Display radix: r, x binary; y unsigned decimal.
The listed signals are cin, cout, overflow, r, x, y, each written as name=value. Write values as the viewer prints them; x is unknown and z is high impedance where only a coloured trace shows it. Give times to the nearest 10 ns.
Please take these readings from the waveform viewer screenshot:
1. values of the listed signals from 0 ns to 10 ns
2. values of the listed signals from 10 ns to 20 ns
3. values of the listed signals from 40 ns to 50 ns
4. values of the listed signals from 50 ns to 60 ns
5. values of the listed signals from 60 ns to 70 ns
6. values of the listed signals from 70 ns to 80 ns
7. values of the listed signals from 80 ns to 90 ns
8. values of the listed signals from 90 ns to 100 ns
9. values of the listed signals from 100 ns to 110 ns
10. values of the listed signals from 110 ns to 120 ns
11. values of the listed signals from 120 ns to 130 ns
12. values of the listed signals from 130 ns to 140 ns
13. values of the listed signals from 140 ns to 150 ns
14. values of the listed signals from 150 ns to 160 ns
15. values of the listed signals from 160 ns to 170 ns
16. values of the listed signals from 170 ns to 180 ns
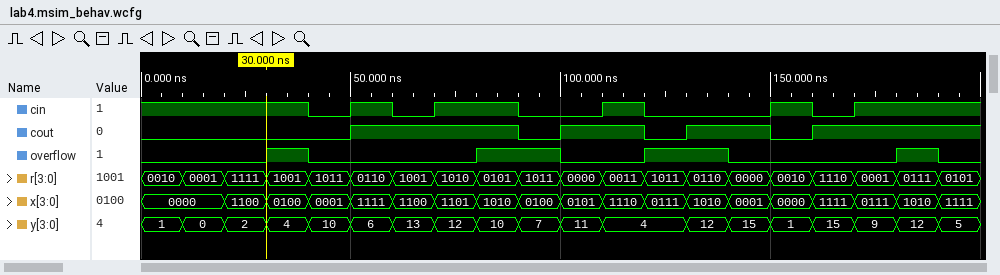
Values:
cin=1, cout=0, overflow=0, r=0010, x=0000, y=1
cin=1, cout=0, overflow=0, r=0001, x=0000, y=0
cin=0, cout=0, overflow=0, r=1011, x=0001, y=10
cin=1, cout=1, overflow=0, r=0110, x=1111, y=6
cin=0, cout=1, overflow=0, r=1001, x=1100, y=13
cin=1, cout=1, overflow=0, r=1010, x=1101, y=12
cin=1, cout=1, overflow=1, r=0101, x=1010, y=10
cin=0, cout=0, overflow=1, r=1011, x=0100, y=7
cin=0, cout=1, overflow=0, r=0000, x=0101, y=11
cin=1, cout=1, overflow=0, r=0011, x=1110, y=4
cin=0, cout=0, overflow=1, r=1011, x=0111, y=4
cin=0, cout=1, overflow=1, r=0110, x=1010, y=12
cin=0, cout=1, overflow=0, r=0000, x=0001, y=15
cin=1, cout=0, overflow=0, r=0010, x=0000, y=1
cin=0, cout=1, overflow=0, r=1110, x=1111, y=15
cin=1, cout=1, overflow=0, r=0001, x=0111, y=9
